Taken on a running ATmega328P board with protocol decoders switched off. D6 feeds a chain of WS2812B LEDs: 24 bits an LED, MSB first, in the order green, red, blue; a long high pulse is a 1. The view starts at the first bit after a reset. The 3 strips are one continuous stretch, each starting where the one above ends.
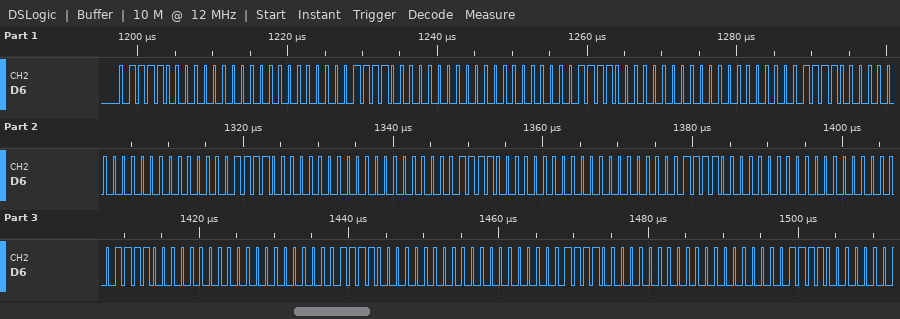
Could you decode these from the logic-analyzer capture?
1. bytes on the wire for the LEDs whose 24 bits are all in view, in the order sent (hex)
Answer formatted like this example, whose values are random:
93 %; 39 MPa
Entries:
78 00 00 78 00 00 78 00 00 78 00 00 78 00 00 78 00 00 78 00 00 78 00 00 78 00 00 78 00 00
